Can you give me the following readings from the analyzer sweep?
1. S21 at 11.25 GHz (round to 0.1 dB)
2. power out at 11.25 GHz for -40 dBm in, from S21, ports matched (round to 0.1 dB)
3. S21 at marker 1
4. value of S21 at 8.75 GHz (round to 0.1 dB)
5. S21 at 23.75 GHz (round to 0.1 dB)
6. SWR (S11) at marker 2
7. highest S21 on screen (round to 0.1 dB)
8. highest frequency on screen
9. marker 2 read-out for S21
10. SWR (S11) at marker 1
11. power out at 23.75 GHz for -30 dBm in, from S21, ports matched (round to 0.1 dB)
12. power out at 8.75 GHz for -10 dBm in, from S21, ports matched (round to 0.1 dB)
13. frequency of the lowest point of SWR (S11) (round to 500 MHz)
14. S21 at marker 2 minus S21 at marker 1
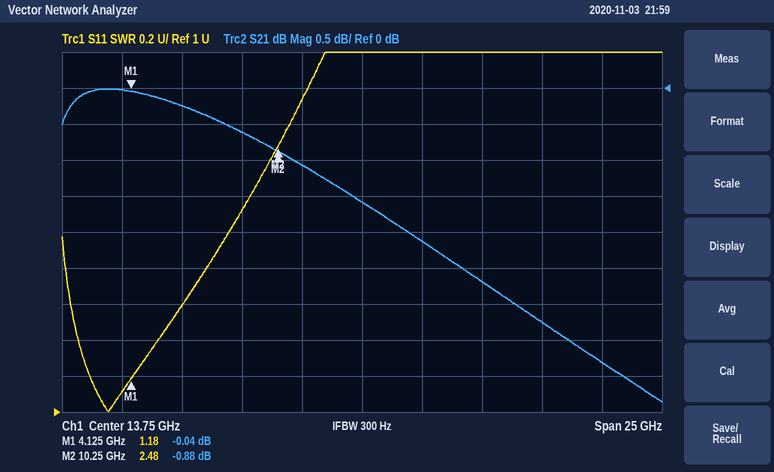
-1.1 dB
-41.1 dBm
-0.04 dB
-0.6 dB
-3.8 dB
2.48
0.0 dB
26.25 GHz
-0.88 dB
1.18
-33.8 dBm
-10.6 dBm
3.0 GHz
-0.84 dB
